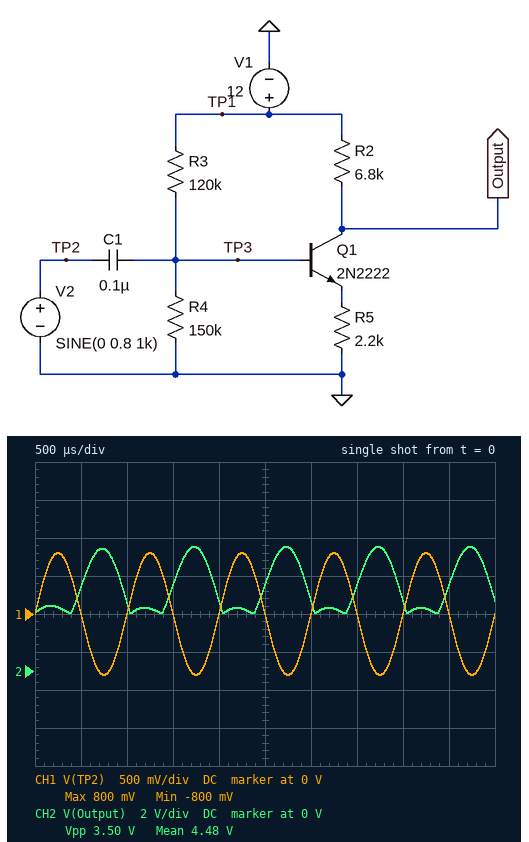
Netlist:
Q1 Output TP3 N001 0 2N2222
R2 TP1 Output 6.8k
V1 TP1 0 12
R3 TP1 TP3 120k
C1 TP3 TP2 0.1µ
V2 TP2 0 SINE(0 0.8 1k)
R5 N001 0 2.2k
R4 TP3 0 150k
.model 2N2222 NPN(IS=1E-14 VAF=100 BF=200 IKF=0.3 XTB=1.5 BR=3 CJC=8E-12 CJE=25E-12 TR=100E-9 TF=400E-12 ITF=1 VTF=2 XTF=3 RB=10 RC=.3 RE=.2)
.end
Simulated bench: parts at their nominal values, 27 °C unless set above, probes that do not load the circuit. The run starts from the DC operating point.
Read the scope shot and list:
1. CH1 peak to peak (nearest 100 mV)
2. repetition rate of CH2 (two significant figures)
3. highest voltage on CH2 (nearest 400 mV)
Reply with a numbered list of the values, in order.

1. 1.6 V
2. 1.0 kHz
3. 6.4 V
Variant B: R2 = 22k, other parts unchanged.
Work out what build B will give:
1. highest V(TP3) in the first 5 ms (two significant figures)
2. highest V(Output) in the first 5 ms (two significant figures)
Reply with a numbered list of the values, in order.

1. 2.3 V
2. 10 V
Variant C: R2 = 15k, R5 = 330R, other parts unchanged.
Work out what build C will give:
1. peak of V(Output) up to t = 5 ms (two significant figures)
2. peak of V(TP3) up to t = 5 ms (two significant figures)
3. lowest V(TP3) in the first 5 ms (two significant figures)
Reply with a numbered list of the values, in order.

1. 12 V
2. 1.1 V
3. -220 mV
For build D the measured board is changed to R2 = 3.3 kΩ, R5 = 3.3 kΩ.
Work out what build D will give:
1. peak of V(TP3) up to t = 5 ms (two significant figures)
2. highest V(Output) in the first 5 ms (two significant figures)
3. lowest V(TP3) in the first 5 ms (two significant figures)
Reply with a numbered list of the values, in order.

1. 6.8 V
2. 7.6 V
3. 5.1 V
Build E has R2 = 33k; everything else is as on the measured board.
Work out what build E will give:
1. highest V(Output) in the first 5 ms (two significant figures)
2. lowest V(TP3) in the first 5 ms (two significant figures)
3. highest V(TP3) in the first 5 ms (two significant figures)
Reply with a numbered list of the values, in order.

1. 12 V
2. 490 mV
3. 2.0 V
